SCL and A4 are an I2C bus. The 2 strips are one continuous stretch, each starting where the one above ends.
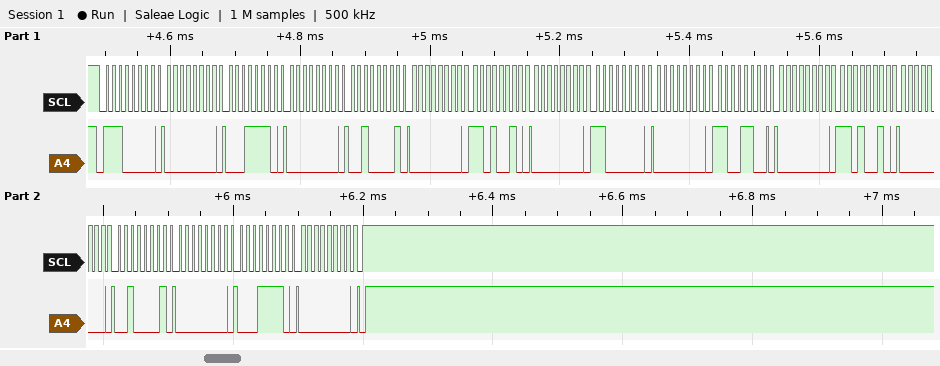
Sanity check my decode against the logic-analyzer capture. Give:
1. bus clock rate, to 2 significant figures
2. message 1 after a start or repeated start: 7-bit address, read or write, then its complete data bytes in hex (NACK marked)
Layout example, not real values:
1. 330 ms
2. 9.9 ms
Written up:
1. 100 kHz
2. 0x70 write: 00 1E 00 21 00 D2 00 C0 00 CC 00 D2 00 21 00 1E 00
